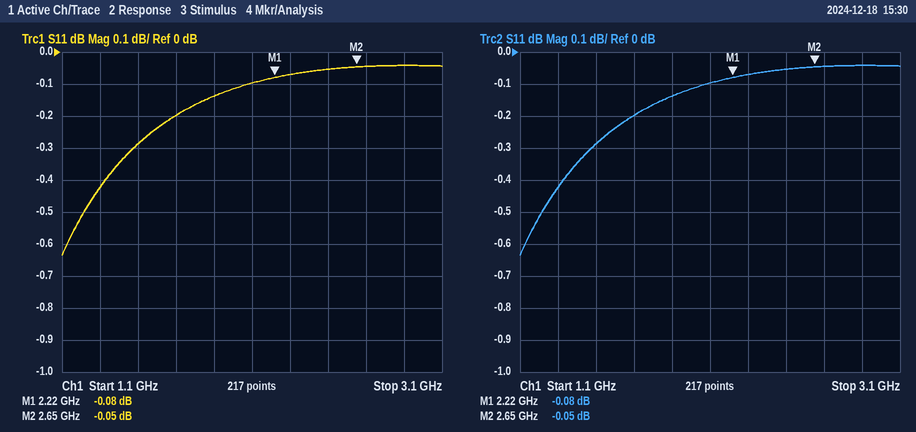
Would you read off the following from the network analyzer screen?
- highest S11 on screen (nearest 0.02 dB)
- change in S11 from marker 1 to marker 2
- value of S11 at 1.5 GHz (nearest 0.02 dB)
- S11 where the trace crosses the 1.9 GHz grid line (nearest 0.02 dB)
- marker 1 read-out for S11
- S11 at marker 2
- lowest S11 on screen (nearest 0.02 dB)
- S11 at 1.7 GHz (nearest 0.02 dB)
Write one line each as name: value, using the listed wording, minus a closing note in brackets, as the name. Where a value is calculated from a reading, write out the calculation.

highest S11 on screen: -0.04 dB
change in S11 from marker 1 to marker 2: -0.05 − (-0.08) = 0.03 dB
value of S11 at 1.5 GHz: -0.28 dB
S11 where the trace crosses the 1.9 GHz grid line: -0.14 dB
marker 1 read-out for S11: -0.08 dB
S11 at marker 2: -0.05 dB
lowest S11 on screen: -0.64 dB
S11 at 1.7 GHz: -0.20 dB
